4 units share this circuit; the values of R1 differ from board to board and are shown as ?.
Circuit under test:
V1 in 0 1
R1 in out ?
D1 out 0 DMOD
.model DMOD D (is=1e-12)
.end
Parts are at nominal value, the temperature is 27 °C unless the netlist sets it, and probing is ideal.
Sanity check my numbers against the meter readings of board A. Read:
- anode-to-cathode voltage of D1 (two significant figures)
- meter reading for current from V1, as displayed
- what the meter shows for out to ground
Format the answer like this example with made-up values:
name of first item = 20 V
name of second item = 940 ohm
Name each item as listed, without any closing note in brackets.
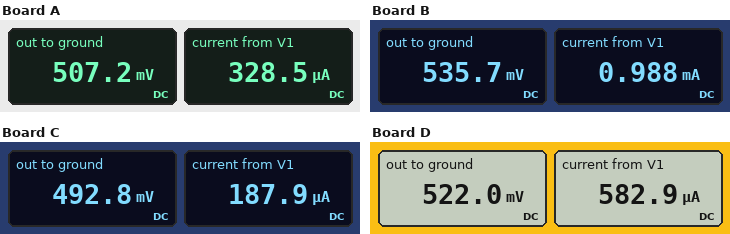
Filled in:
anode-to-cathode voltage of D1 = 510 mV
meter reading for current from V1, as displayed = 328.5 µA
what the meter shows for out to ground = 507.2 mV
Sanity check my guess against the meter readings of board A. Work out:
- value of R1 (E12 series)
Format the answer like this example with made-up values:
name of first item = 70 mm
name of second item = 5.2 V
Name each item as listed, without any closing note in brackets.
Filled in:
value of R1 = 1.5 kΩ
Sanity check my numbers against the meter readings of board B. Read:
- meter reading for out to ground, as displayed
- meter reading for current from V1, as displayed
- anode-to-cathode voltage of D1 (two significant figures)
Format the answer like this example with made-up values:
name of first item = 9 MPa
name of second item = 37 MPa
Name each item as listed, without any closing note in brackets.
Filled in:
meter reading for out to ground, as displayed = 535.7 mV
meter reading for current from V1, as displayed = 0.988 mA
anode-to-cathode voltage of D1 = 540 mV
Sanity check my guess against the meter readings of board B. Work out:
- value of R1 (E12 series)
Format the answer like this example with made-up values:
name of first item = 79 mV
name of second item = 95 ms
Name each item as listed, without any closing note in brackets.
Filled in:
value of R1 = 470 Ω
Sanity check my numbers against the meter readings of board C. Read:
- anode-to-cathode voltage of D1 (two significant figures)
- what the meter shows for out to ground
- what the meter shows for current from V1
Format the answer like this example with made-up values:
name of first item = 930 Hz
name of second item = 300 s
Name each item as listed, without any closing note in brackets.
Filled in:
anode-to-cathode voltage of D1 = 490 mV
what the meter shows for out to ground = 492.8 mV
what the meter shows for current from V1 = 187.9 µA
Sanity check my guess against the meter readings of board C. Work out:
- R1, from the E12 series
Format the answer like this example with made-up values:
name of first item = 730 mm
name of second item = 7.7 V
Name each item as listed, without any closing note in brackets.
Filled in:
R1, from the E12 series = 2.7 kΩ
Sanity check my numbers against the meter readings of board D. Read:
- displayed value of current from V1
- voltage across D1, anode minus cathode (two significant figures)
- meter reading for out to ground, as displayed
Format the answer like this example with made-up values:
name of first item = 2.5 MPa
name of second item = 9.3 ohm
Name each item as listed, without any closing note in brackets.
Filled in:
displayed value of current from V1 = 582.9 µA
voltage across D1, anode minus cathode = 520 mV
meter reading for out to ground, as displayed = 522.0 mV
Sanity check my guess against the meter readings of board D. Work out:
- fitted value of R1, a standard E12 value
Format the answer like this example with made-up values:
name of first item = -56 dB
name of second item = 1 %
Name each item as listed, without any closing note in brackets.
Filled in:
fitted value of R1, a standard E12 value = 820 Ω
